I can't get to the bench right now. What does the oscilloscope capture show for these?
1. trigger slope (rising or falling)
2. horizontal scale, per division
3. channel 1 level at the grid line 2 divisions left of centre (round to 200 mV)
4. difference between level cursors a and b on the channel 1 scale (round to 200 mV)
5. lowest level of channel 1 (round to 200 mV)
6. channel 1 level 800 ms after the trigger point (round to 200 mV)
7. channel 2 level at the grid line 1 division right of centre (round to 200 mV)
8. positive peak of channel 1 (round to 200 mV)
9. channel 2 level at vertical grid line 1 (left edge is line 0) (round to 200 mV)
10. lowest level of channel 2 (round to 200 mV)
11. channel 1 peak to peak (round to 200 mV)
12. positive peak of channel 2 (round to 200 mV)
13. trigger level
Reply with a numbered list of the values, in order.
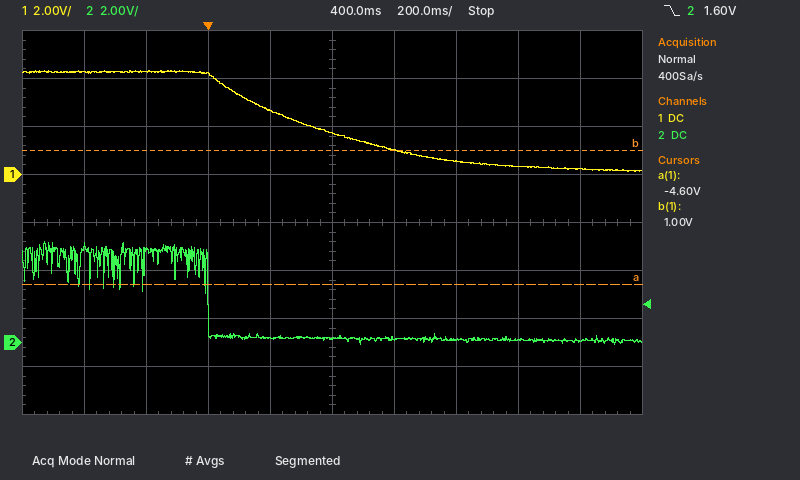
1. falling
2. 200 ms
3. 4.2 V
4. 5.6 V
5. 200 mV
6. 600 mV
7. 200 mV
8. 4.4 V
9. 4.0 V
10. 0.0 V
11. 4.2 V
12. 4.2 V
13. 1.60 V
